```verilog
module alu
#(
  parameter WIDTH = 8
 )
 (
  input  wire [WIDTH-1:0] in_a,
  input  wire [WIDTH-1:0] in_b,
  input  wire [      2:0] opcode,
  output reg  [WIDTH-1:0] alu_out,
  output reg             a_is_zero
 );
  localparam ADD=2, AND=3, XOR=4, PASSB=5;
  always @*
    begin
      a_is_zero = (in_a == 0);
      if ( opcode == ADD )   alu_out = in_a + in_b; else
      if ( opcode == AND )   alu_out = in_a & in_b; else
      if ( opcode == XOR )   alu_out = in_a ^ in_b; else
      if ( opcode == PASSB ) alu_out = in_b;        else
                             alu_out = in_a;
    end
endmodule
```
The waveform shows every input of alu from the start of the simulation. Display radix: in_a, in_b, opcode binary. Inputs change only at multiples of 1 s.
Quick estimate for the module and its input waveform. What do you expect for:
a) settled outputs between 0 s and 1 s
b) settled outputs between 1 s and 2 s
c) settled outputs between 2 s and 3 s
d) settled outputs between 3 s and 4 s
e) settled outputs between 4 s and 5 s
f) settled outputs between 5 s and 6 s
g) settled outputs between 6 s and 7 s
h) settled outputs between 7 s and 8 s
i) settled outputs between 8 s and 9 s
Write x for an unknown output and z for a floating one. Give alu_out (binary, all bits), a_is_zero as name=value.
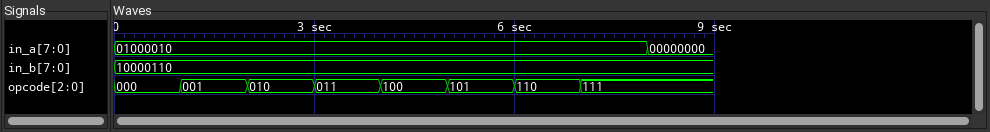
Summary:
alu_out=01000010, a_is_zero=0
alu_out=01000010, a_is_zero=0
alu_out=11001000, a_is_zero=0
alu_out=00000010, a_is_zero=0
alu_out=11000100, a_is_zero=0
alu_out=10000110, a_is_zero=0
alu_out=01000010, a_is_zero=0
alu_out=01000010, a_is_zero=0
alu_out=00000000, a_is_zero=1
